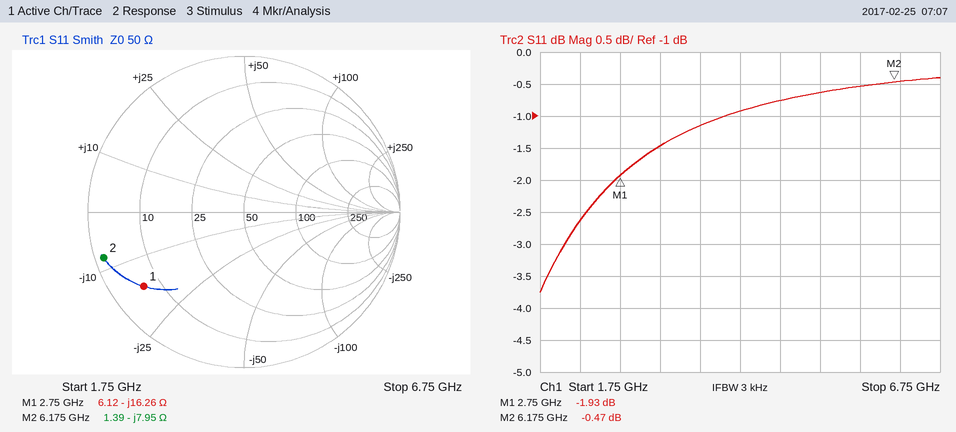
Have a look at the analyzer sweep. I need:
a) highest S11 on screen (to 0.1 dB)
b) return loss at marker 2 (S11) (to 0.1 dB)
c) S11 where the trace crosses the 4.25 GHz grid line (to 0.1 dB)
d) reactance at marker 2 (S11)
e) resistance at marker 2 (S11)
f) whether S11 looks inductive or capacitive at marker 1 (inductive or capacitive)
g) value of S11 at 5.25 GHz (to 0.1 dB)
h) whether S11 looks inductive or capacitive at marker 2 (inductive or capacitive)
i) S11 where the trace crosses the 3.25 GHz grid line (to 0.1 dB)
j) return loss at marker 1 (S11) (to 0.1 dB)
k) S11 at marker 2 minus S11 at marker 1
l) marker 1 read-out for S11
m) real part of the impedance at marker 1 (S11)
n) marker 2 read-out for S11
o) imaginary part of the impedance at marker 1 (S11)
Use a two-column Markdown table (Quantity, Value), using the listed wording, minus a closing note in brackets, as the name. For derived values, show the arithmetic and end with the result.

| Quantity | Value |
|---|---|
| highest S11 on screen | -0.4 dB |
| return loss at marker 2 (S11) | 0.5 dB |
| S11 where the trace crosses the 4.25 GHz grid line | -0.9 dB |
| reactance at marker 2 | -7.95 Ω |
| resistance at marker 2 | 1.39 Ω |
| whether S11 looks inductive or capacitive at marker 1 | capacitive |
| value of S11 at 5.25 GHz | -0.6 dB |
| whether S11 looks inductive or capacitive at marker 2 | capacitive |
| S11 where the trace crosses the 3.25 GHz grid line | -1.5 dB |
| return loss at marker 1 (S11) | 1.9 dB |
| S11 at marker 2 minus S11 at marker 1 | -0.47 − (-1.93) = 1.46 dB |
| marker 1 read-out for S11 | -1.93 dB |
| real part of the impedance at marker 1 | 6.12 Ω |
| marker 2 read-out for S11 | -0.47 dB |
| imaginary part of the impedance at marker 1 | -16.26 Ω |
